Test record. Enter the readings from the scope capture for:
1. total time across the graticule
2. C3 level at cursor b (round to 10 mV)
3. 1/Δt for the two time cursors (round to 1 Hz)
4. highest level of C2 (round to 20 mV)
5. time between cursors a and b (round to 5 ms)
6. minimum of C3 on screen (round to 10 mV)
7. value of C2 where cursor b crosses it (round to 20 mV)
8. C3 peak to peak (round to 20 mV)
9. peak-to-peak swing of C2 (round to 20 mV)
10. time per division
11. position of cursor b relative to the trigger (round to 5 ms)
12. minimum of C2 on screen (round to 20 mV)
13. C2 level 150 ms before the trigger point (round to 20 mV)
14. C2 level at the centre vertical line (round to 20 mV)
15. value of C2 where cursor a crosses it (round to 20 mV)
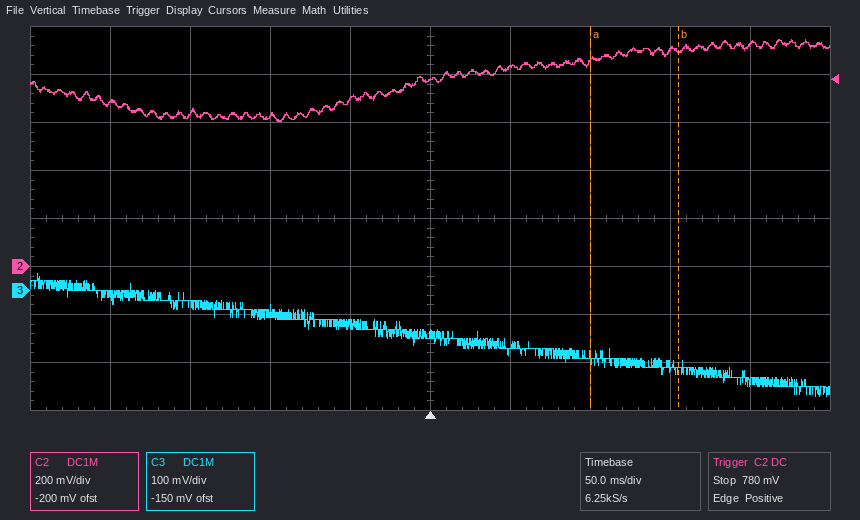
500 ms
-170 mV
18 Hz
940 mV
55 ms
-220 mV
900 mV
260 mV
340 mV
50 ms
+155 ms
600 mV
640 mV
780 mV
860 mV
